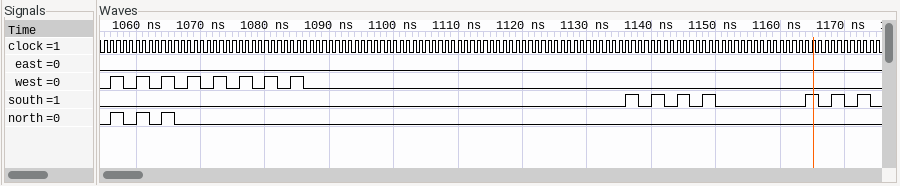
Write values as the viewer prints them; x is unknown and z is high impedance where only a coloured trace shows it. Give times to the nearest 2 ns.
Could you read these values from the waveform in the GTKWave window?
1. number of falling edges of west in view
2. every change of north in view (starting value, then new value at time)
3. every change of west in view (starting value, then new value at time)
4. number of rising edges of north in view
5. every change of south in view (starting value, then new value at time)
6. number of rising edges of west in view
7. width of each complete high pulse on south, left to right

8
0, 1 at 1056 ns, 0 at 1058 ns, 1 at 1060 ns, 0 at 1062 ns, 1 at 1064 ns, 0 at 1066 ns
0, 1 at 1056 ns, 0 at 1058 ns, 1 at 1060 ns, 0 at 1062 ns, 1 at 1064 ns, 0 at 1066 ns, 1 at 1068 ns, 0 at 1070 ns, 1 at 1072 ns, 0 at 1074 ns, 1 at 1076 ns, 0 at 1078 ns, 1 at 1080 ns, 0 at 1082 ns, 1 at 1084 ns, 0 at 1086 ns
3
0, 1 at 1136 ns, 0 at 1138 ns, 1 at 1140 ns, 0 at 1142 ns, 1 at 1144 ns, 0 at 1146 ns, 1 at 1148 ns, 0 at 1150 ns, 1 at 1164 ns, 0 at 1166 ns, 1 at 1168 ns, 0 at 1170 ns, 1 at 1172 ns, 0 at 1174 ns
8
2 ns, 2 ns, 2 ns, 2 ns, 2 ns, 2 ns, 2 ns
